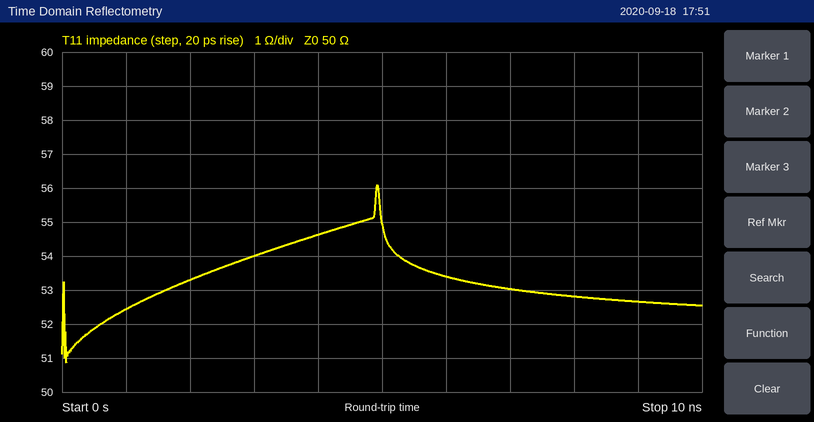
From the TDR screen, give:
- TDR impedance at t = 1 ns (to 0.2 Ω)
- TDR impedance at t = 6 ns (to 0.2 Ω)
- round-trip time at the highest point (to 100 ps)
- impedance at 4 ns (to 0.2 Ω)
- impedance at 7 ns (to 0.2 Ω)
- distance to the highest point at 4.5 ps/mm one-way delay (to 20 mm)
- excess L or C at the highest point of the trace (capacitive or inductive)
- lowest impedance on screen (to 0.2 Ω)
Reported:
52.4 Ω
53.4 Ω
4.9 ns
54.6 Ω
53.0 Ω
540 mm
inductive
50.8 Ω
